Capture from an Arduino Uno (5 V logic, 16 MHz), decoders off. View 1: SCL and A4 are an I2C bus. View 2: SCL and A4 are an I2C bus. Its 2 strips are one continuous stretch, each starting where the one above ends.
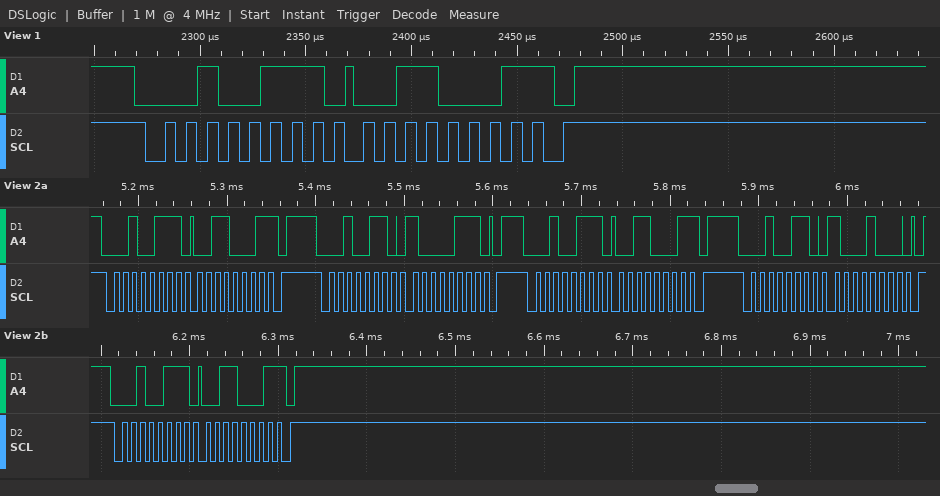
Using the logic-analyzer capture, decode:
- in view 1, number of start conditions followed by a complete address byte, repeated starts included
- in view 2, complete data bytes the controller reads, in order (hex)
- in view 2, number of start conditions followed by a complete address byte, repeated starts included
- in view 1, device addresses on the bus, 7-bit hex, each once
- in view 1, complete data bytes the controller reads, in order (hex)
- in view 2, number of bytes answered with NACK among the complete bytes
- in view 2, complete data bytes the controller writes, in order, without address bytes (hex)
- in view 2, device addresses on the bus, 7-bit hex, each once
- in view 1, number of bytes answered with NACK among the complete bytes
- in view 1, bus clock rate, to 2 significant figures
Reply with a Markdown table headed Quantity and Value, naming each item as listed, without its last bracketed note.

| Quantity | Value |
|---|---|
| in view 1, number of start conditions followed by a complete address byte, repeated starts included | 1 |
| in view 2, complete data bytes the controller reads, in order | 31 31 31 |
| in view 2, number of start conditions followed by a complete address byte, repeated starts included | 5 |
| in view 1, device addresses on the bus, 7-bit hex, each once | 0x13 |
| in view 1, complete data bytes the controller reads, in order | 31 |
| in view 2, number of bytes answered with NACK among the complete bytes | 3 |
| in view 2, complete data bytes the controller writes, in order, without address bytes | 87 88 |
| in view 2, device addresses on the bus, 7-bit hex, each once | 0x13 |
| in view 1, number of bytes answered with NACK among the complete bytes | 1 |
| in view 1, bus clock rate, to 2 significant figures | 100 kHz |
